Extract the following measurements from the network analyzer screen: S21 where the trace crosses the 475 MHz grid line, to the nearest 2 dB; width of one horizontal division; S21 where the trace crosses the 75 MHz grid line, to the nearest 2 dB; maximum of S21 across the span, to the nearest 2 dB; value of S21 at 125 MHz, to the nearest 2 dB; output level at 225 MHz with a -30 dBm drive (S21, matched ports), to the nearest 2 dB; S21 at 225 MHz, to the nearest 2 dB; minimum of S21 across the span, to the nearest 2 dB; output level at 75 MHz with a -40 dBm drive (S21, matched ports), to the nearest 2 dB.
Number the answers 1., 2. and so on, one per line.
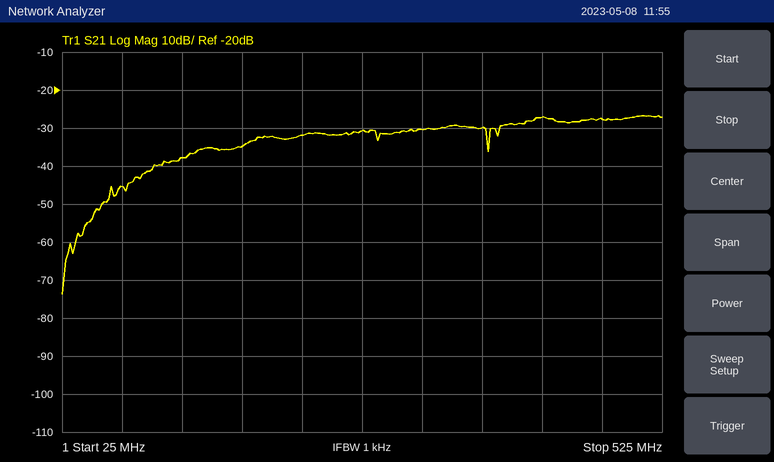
1. -28 dB
2. 50 MHz
3. -46 dB
4. -26 dB
5. -38 dB
6. -62 dBm
7. -32 dB
8. -74 dB
9. -86 dBm
